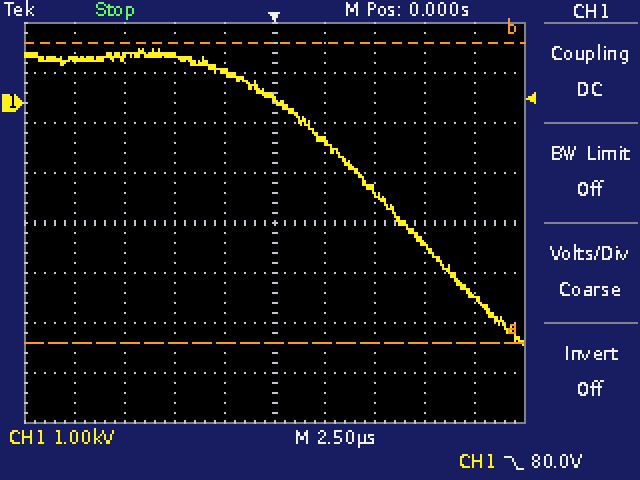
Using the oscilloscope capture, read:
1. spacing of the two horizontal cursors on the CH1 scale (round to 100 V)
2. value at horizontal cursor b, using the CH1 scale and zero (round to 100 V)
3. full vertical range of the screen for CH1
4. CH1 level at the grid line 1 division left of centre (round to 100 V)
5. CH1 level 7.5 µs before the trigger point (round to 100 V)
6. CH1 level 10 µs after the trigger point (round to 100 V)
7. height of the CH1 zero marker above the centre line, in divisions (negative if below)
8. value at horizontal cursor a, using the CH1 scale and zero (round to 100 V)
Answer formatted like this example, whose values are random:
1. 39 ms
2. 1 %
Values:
1. 6.0 kV
2. 1.2 kV
3. 8 kV
4. 600 V
5. 900 V
6. -3.9 kV
7. +2.4 div
8. -4.8 kV
